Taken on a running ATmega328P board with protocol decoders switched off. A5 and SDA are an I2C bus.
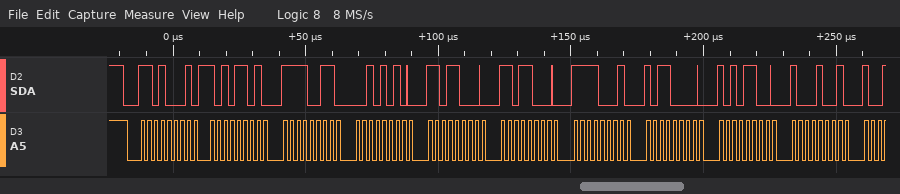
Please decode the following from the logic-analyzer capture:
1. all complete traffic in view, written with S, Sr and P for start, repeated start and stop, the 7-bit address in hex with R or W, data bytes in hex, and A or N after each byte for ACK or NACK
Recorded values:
S 68R A AD A F3 A 2A A D8 A D8 A F1 A B0 A AC A 89 A
